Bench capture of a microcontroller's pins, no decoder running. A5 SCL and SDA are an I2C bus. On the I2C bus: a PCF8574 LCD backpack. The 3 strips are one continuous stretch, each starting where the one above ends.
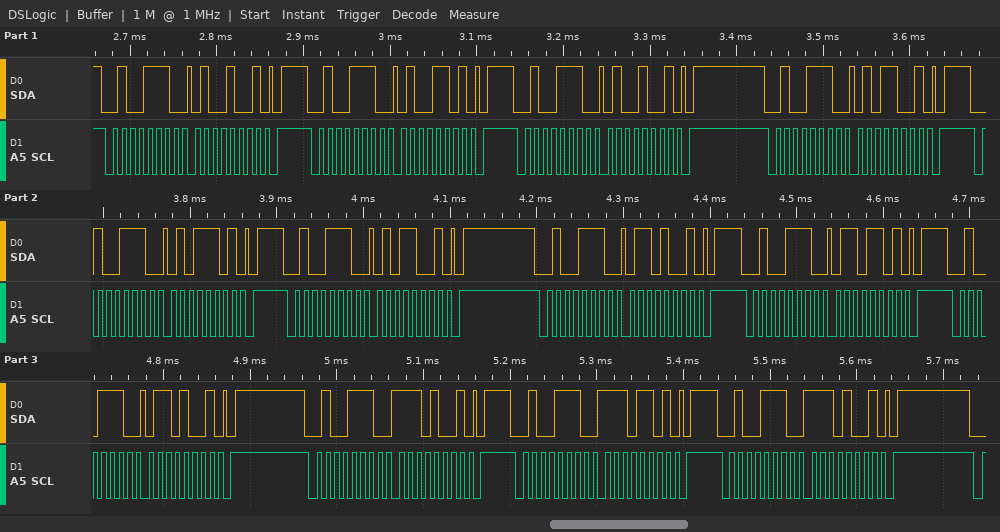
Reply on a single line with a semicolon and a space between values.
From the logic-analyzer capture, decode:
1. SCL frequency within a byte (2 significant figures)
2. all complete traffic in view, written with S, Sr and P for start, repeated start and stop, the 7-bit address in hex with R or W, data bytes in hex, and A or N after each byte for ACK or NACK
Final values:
100 kHz; S 27W A 49 A P S 27W A 4D A P S 27W A 49 A P S 27W A 59 A P S 27W A 5D A P S 27W A 59 A P S 27W A 69 A P S 27W A 6D A P S 27W A 69 A P S 27W A E9 A P S 27W A ED A P S 27W A E9 A P
